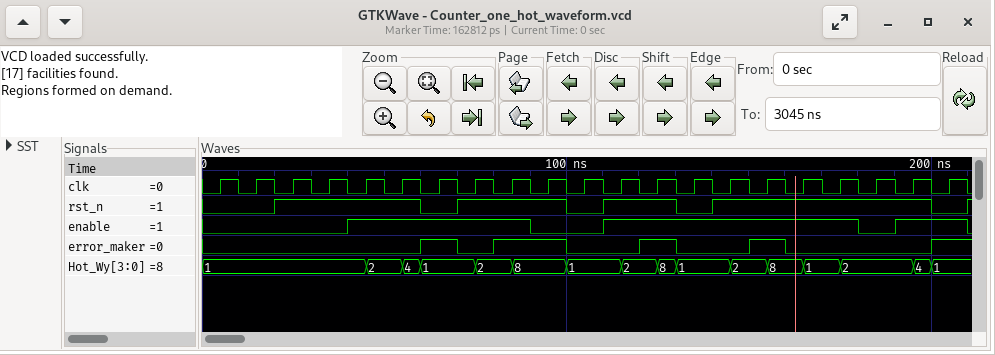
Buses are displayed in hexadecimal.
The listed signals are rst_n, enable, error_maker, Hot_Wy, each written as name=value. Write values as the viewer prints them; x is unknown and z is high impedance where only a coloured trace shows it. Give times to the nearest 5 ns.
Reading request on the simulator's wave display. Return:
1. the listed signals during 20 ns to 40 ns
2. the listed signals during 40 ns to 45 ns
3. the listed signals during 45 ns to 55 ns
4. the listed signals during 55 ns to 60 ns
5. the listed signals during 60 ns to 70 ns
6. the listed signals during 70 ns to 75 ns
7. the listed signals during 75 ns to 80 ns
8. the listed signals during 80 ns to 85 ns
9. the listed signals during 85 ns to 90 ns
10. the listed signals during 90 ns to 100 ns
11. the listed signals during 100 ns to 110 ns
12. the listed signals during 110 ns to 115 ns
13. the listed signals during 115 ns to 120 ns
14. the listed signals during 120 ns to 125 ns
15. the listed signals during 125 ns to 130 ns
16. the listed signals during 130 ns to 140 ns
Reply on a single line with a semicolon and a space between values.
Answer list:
rst_n=1, enable=0, error_maker=0, Hot_Wy=1; rst_n=1, enable=1, error_maker=0, Hot_Wy=1; rst_n=1, enable=1, error_maker=0, Hot_Wy=2; rst_n=1, enable=1, error_maker=0, Hot_Wy=4; rst_n=0, enable=1, error_maker=1, Hot_Wy=1; rst_n=1, enable=1, error_maker=0, Hot_Wy=1; rst_n=1, enable=1, error_maker=0, Hot_Wy=2; rst_n=1, enable=1, error_maker=1, Hot_Wy=2; rst_n=1, enable=1, error_maker=1, Hot_Wy=8; rst_n=1, enable=0, error_maker=1, Hot_Wy=8; rst_n=0, enable=0, error_maker=0, Hot_Wy=1; rst_n=1, enable=1, error_maker=0, Hot_Wy=1; rst_n=1, enable=1, error_maker=0, Hot_Wy=2; rst_n=1, enable=1, error_maker=1, Hot_Wy=2; rst_n=1, enable=1, error_maker=1, Hot_Wy=8; rst_n=0, enable=1, error_maker=0, Hot_Wy=1
